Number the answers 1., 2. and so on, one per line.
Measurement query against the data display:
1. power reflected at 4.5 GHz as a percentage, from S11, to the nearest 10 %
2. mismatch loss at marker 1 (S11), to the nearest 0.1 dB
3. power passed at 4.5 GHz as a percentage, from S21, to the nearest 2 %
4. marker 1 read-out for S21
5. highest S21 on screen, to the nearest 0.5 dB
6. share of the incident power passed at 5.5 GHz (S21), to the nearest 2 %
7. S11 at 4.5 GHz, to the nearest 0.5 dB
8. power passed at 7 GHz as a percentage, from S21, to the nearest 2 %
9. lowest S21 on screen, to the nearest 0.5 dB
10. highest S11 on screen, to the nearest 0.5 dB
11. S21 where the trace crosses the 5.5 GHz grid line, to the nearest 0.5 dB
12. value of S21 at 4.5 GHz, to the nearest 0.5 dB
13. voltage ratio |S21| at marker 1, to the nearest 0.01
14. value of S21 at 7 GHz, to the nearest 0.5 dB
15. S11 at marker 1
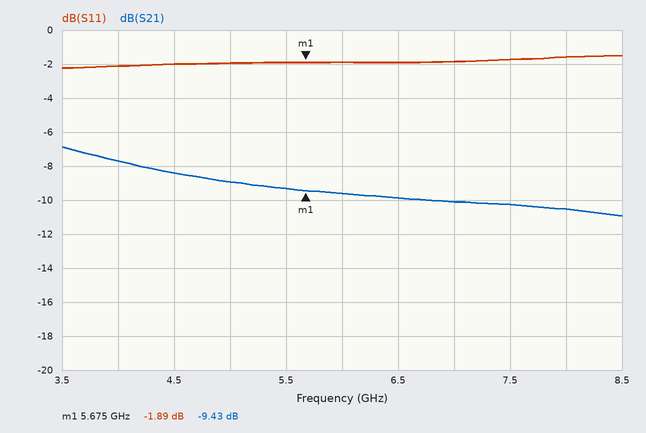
1. 60 %
2. 4.5 dB
3. 14 %
4. -9.43 dB
5. -7.0 dB
6. 12 %
7. -2.0 dB
8. 10 %
9. -11.0 dB
10. -1.5 dB
11. -9.5 dB
12. -8.5 dB
13. 0.34
14. -10.0 dB
15. -1.89 dB
